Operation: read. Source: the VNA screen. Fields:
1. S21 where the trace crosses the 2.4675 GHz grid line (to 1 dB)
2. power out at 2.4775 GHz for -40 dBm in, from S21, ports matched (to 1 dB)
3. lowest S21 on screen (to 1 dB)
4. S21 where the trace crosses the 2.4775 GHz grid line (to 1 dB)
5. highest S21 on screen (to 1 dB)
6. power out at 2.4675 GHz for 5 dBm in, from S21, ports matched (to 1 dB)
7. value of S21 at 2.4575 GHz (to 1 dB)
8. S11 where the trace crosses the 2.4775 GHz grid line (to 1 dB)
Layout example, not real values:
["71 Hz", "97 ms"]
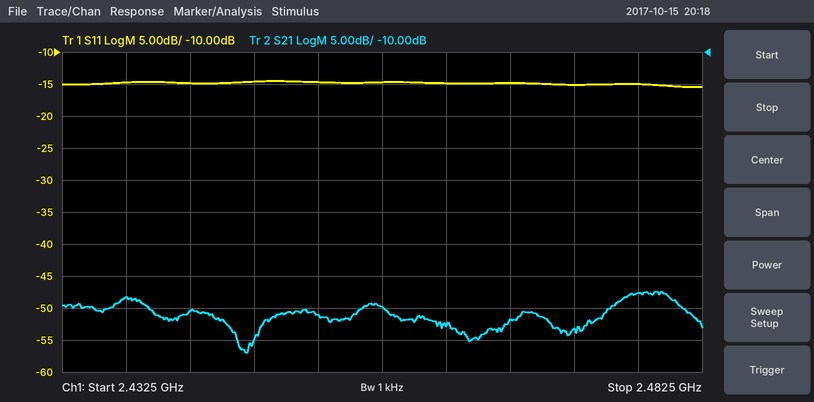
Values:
["-52 dB", "-88 dBm", "-57 dB", "-48 dB", "-47 dB", "-47 dBm", "-50 dB", "-15 dB"]
